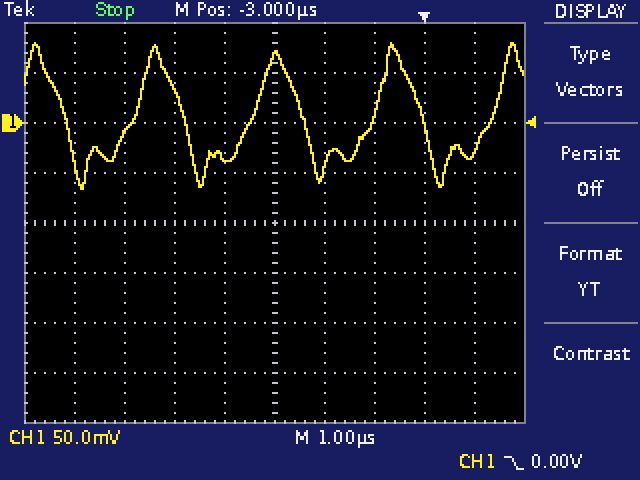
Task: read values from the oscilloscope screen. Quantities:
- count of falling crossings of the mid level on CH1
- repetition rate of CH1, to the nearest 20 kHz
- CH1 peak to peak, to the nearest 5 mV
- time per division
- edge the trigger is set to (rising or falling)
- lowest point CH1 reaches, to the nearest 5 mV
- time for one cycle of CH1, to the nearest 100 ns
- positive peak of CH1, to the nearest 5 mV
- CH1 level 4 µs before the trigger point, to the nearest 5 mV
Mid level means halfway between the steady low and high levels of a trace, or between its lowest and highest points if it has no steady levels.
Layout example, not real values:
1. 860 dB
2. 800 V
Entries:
1. 4
2. 420 kHz
3. 145 mV
4. 1 µs
5. falling
6. -65 mV
7. 2.4 µs
8. 80 mV
9. -35 mV
